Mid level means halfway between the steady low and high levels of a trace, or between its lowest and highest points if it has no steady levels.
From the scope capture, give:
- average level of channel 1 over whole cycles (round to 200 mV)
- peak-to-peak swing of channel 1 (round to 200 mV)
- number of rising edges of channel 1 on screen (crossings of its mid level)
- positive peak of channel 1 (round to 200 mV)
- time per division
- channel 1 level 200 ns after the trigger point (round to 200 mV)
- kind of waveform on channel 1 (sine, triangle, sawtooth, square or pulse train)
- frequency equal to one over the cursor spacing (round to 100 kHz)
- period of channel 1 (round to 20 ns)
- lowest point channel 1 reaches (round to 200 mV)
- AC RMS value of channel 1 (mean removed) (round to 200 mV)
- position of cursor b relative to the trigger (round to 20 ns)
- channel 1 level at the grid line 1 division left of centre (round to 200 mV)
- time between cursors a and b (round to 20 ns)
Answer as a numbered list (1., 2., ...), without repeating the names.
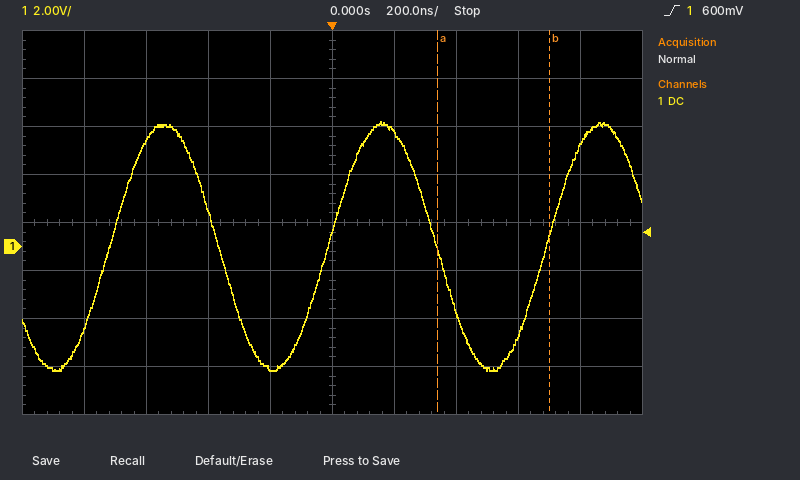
1. 0.0 V
2. 10.4 V
3. 3
4. 5.2 V
5. 200 ns
6. 4.8 V
7. sine
8. 2.8 MHz
9. 700 ns
10. -5.2 V
11. 3.6 V
12. +700 ns
13. -5.0 V
14. 360 ns
